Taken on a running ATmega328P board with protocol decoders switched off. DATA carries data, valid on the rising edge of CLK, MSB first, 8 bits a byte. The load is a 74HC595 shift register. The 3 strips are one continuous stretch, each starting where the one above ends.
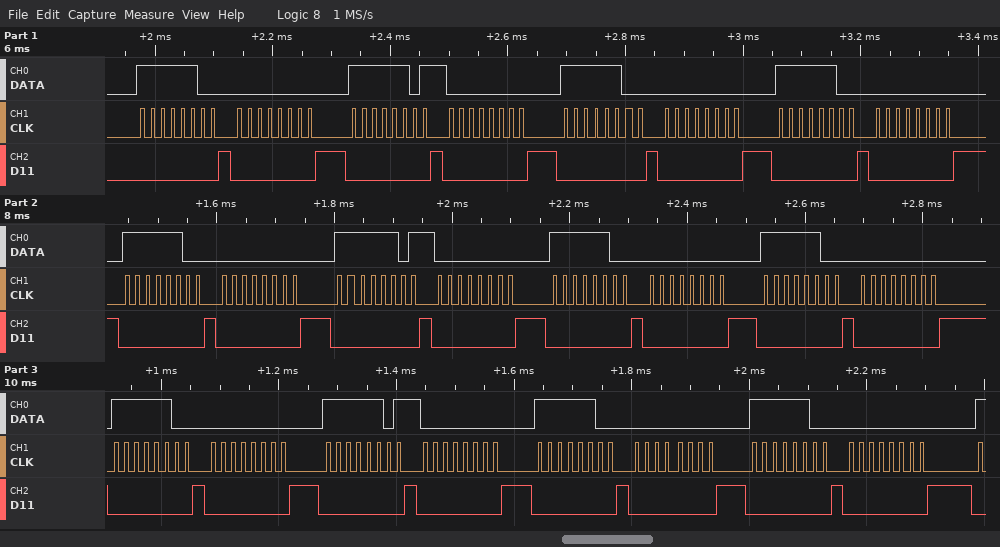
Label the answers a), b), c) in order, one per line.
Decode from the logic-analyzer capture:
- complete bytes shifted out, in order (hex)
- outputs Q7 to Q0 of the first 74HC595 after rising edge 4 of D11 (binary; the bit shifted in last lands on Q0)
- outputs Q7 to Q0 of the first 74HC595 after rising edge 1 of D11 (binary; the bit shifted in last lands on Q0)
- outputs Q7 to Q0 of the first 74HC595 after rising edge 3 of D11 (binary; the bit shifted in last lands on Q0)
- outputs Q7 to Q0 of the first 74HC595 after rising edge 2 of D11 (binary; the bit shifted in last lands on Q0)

a) FC 00 FD 00 FC 00 FC 00 FC 00 FD 00 FC 00 FC 00 FC 00 FD 00 FC 00 FC 00
b) 00000000
c) 11111100
d) 11111101
e) 00000000
